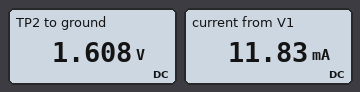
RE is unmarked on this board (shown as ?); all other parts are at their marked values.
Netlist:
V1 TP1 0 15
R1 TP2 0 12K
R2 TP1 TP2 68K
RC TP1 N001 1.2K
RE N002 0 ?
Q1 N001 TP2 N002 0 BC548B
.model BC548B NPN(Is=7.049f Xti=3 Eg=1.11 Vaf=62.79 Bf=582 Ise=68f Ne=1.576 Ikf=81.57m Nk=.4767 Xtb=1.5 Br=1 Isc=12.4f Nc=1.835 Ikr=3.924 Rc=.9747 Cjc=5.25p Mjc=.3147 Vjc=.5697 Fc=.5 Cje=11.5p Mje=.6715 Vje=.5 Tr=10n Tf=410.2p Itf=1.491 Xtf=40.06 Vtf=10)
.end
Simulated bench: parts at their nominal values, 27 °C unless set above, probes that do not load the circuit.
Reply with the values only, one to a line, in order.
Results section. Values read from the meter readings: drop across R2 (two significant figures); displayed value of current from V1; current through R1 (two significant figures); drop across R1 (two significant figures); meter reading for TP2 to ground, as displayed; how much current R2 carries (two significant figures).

13 V
11.83 mA
130 µA
1.6 V
1.608 V
200 µA
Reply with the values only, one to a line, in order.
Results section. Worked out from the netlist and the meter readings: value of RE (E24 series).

75 Ω
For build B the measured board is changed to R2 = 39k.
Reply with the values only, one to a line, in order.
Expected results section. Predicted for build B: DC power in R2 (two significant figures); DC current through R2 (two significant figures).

4.6 mW
340 µA
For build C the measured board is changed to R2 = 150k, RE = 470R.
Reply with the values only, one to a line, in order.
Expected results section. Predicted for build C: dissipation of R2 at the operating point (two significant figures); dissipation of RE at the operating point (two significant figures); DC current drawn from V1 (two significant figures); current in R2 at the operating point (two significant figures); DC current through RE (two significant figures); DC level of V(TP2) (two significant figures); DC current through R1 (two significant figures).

1.3 mW
400 µW
1.0 mA
93 µA
920 µA
1.1 V
91 µA
